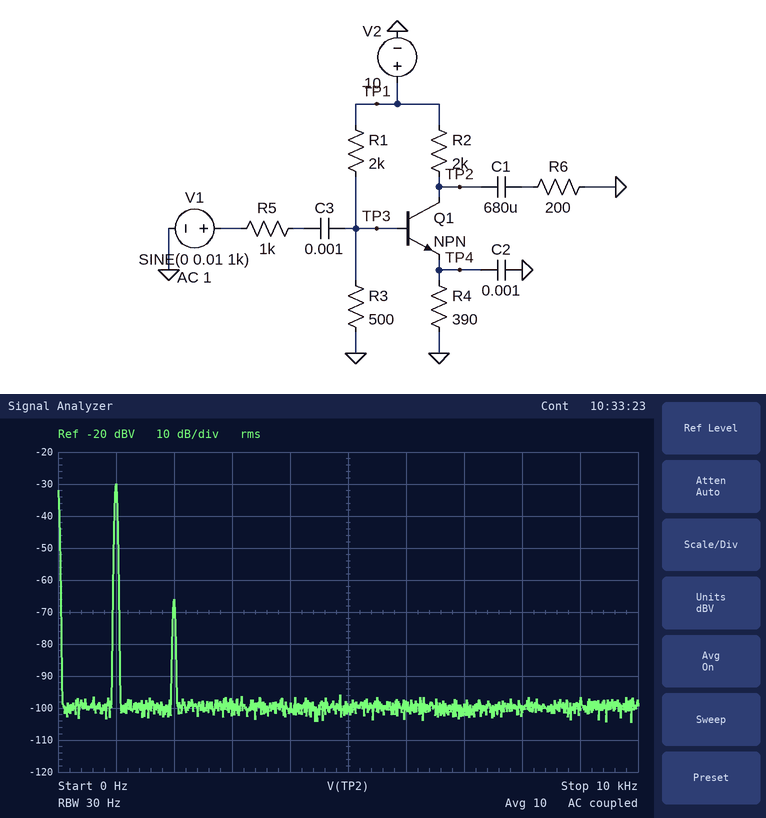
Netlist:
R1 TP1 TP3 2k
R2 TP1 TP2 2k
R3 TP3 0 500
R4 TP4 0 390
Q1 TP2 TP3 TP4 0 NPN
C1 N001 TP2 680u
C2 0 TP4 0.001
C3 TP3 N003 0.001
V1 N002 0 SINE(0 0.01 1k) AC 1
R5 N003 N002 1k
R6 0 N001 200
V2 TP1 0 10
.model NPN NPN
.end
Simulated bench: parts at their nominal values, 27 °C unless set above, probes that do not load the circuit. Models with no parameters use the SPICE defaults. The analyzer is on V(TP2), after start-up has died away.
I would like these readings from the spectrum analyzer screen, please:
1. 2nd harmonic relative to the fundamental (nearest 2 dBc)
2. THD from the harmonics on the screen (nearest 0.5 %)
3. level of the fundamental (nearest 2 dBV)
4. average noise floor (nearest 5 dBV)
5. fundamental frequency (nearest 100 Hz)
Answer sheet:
-36 dBc
1.5 %
-30 dBV
-100 dBV
1.0 kHz
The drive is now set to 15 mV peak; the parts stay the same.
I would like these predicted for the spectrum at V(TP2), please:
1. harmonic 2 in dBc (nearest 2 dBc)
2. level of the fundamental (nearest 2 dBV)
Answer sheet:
-32 dBc
-26 dBV
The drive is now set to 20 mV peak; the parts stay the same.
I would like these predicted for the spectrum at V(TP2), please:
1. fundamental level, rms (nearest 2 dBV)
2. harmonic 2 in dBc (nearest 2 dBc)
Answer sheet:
-24 dBV
-30 dBc
